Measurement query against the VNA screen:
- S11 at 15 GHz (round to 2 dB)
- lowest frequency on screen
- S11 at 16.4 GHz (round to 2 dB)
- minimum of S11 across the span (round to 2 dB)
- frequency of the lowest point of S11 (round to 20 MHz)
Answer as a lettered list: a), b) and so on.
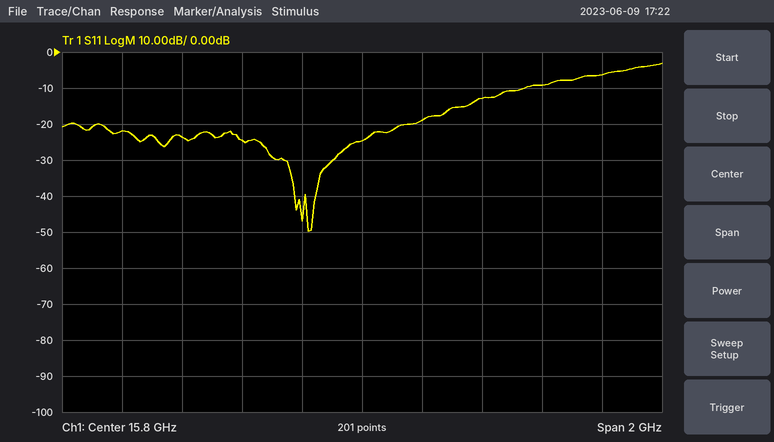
a) -22 dB
b) 14.8 GHz
c) -10 dB
d) -50 dB
e) 15.62 GHz
